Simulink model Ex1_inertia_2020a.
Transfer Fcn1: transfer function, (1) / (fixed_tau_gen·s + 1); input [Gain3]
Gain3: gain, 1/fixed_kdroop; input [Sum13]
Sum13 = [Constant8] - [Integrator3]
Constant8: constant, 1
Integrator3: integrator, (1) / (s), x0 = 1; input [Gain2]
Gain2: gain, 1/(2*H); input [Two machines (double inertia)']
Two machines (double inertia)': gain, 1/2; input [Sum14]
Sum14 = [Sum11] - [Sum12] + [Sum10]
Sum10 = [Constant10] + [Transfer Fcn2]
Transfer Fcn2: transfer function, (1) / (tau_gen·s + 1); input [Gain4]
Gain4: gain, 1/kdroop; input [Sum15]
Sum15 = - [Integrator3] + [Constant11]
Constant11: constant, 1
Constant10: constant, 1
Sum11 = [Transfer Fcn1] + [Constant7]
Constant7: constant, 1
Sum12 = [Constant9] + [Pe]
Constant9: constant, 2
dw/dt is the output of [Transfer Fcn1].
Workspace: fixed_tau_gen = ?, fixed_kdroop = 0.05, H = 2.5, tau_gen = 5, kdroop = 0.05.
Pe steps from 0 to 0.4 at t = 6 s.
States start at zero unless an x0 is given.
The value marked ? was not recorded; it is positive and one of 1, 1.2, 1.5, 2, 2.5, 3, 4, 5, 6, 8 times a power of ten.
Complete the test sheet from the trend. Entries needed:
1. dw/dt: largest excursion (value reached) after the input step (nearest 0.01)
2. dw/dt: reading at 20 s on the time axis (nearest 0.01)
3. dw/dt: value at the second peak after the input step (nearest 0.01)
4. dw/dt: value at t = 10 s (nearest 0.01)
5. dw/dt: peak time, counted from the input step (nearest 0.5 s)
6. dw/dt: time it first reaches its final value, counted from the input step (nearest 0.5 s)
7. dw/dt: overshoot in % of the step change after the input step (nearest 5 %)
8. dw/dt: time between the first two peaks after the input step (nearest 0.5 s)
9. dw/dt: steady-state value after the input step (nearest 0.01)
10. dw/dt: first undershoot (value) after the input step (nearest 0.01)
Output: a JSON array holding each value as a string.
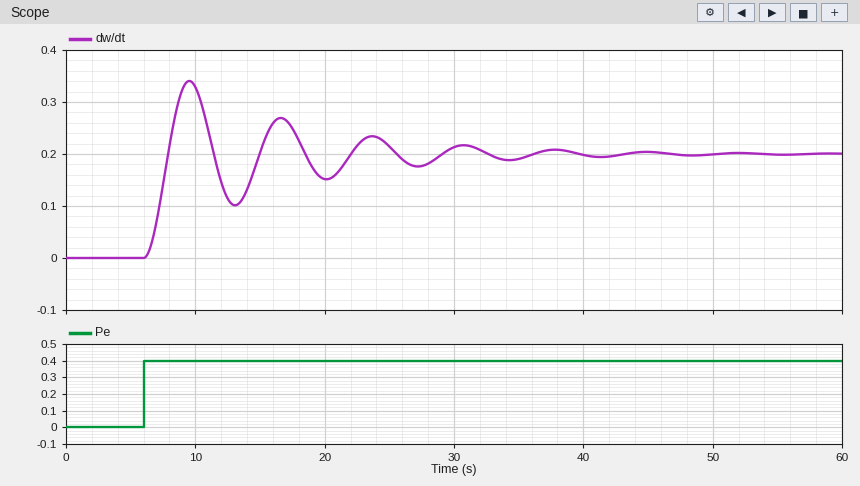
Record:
["0.34", "0.15", "0.27", "0.33", "3.5 s", "2.0 s", "70 %", "7.0 s", "0.20", "0.10"]
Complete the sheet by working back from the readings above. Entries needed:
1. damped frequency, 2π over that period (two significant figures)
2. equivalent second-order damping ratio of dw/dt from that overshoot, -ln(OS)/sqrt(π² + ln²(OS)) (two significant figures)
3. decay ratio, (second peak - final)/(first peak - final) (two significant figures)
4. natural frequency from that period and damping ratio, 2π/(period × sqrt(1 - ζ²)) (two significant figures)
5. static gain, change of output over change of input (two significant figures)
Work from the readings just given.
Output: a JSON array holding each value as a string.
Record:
["0.90 rad/s", "0.11", "0.50", "0.90 rad/s", "0.50"]
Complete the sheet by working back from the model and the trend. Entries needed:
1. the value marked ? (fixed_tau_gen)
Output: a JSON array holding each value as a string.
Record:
["5"]
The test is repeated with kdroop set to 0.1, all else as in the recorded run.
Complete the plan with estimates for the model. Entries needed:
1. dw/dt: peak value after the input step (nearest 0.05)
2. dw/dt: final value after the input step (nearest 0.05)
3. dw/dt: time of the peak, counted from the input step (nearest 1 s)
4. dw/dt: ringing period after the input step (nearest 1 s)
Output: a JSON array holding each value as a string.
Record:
["0.45", "0.25", "4 s", "8 s"]
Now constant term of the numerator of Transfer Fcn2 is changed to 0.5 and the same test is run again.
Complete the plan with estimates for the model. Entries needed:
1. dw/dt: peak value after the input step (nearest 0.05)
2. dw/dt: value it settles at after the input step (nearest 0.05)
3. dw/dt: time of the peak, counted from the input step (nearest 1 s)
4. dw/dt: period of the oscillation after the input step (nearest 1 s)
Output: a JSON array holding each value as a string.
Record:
["0.45", "0.25", "4 s", "8 s"]
